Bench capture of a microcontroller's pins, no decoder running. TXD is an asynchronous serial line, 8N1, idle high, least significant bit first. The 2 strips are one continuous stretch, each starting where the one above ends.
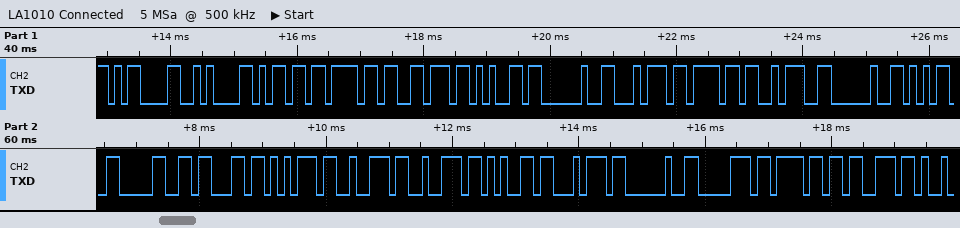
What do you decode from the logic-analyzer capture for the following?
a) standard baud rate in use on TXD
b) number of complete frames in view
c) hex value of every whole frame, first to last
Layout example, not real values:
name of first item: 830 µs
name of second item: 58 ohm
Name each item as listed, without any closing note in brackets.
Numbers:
standard baud rate in use on TXD: 9600 baud
number of complete frames in view: 23
hex value of every whole frame, first to last: 0D 0A 6D 6F 76 65 20 74 6F 3A 20 35 30 63 75 72 72 65 74 20 70 6F 73
